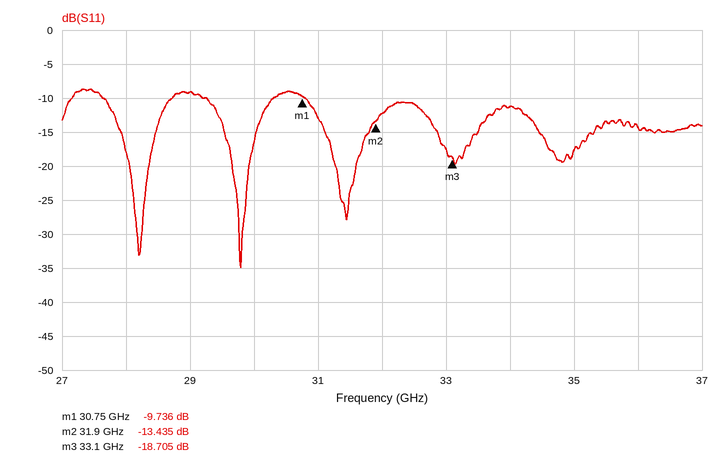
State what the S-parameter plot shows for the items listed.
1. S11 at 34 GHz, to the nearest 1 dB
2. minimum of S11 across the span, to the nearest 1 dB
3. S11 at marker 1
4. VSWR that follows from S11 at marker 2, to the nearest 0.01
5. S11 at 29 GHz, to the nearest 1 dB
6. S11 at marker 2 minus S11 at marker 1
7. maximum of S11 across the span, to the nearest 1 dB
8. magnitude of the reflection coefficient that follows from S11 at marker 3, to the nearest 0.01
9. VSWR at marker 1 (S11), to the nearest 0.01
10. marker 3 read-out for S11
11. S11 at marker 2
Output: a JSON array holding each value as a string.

["-11 dB", "-35 dB", "-9.736 dB", "1.54", "-9 dB", "-3.699 dB", "-9 dB", "0.12", "1.97", "-18.705 dB", "-13.435 dB"]
